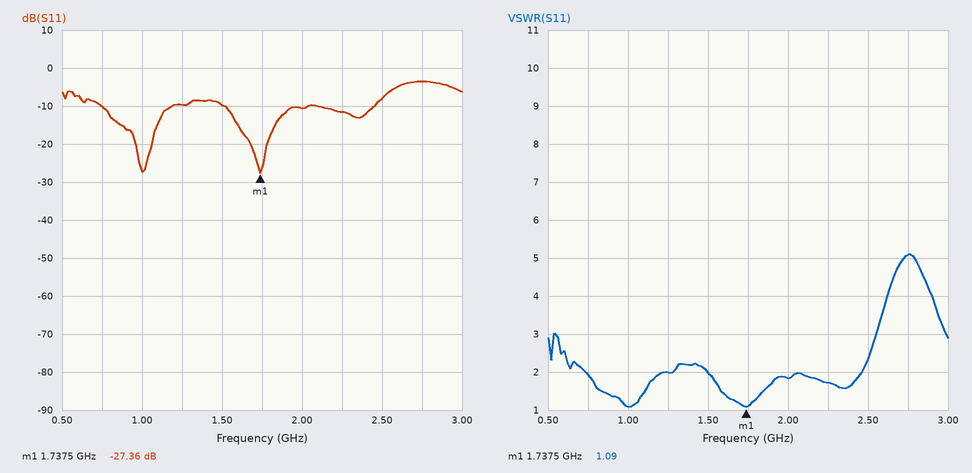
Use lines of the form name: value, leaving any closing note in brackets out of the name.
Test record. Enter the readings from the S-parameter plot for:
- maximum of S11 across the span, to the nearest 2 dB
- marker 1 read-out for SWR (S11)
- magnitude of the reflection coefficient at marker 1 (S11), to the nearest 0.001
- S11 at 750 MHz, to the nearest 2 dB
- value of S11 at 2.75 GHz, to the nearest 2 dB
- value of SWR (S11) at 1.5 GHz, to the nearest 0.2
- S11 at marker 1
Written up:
maximum of S11 across the span, to the nearest 2 dB: -4 dB
marker 1 read-out for SWR: 1.09
magnitude of the reflection coefficient at marker 1 (S11), to the nearest 0.001: 0.043
S11 at 750 MHz, to the nearest 2 dB: -10 dB
value of S11 at 2.75 GHz, to the nearest 2 dB: -4 dB
value of SWR (S11) at 1.5 GHz, to the nearest 0.2: 2.0
S11 at marker 1: -27.36 dB
